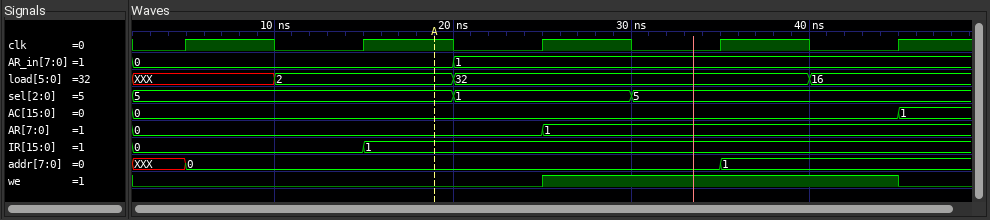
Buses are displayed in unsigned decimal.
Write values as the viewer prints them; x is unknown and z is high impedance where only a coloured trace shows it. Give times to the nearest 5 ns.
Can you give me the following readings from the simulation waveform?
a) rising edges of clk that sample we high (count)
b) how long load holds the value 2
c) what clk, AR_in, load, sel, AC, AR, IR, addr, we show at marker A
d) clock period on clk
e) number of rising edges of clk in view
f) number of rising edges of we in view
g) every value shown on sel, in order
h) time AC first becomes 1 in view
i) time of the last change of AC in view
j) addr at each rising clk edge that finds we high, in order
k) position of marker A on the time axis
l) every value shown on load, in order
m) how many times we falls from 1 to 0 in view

2
10 ns
clk=1, AR_in=0, load=2, sel=5, AC=0, AR=0, IR=1, addr=0, we=0
10 ns
5
1
5, 1, 5
45 ns
45 ns
0, 1
20 ns
XXX, 2, 32, 16
1
